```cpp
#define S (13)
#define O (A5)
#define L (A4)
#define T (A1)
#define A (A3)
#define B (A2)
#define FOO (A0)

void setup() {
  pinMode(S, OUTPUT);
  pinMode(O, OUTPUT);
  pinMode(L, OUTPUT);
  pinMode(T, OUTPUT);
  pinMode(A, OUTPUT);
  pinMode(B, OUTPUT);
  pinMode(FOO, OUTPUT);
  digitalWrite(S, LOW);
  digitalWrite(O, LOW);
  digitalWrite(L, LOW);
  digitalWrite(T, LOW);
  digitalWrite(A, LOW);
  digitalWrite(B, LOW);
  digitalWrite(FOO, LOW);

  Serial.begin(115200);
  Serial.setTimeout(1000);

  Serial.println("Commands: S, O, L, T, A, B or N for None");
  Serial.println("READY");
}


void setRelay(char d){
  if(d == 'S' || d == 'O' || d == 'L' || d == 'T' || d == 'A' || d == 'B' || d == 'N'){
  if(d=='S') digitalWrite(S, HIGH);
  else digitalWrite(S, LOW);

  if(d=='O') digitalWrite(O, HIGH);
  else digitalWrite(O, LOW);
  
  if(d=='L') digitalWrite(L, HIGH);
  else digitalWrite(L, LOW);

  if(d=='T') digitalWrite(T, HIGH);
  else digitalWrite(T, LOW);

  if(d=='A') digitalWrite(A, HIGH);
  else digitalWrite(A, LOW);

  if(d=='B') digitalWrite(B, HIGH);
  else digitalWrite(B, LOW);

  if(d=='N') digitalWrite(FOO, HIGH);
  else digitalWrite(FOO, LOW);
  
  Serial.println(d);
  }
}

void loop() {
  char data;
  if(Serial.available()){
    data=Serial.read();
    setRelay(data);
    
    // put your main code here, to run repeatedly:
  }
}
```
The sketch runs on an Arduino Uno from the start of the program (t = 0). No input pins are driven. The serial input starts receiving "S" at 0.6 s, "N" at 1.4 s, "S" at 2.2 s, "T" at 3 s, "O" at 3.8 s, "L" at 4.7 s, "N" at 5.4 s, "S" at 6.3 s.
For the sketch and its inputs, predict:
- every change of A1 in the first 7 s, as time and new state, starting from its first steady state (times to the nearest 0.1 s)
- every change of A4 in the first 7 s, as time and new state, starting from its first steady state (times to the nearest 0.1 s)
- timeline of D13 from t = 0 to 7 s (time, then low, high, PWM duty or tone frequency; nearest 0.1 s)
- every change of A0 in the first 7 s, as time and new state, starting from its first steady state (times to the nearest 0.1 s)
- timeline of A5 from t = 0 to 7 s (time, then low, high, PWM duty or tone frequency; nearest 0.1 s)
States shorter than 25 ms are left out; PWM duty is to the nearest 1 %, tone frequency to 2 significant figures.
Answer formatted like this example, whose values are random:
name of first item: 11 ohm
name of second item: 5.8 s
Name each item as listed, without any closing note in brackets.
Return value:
every change of A1 in the first 7 s, as time and new state, starting from its first steady state: 0 s low; 3 s high; 3.8 s low
every change of A4 in the first 7 s, as time and new state, starting from its first steady state: 0 s low; 4.7 s high; 5.4 s low
timeline of D13 from t = 0 to 7 s: 0 s low; 0.6 s high; 1.4 s low; 2.2 s high; 3 s low; 6.3 s high
every change of A0 in the first 7 s, as time and new state, starting from its first steady state: 0 s low; 1.4 s high; 2.2 s low; 5.4 s high; 6.3 s low
timeline of A5 from t = 0 to 7 s: 0 s low; 3.8 s high; 4.7 s low
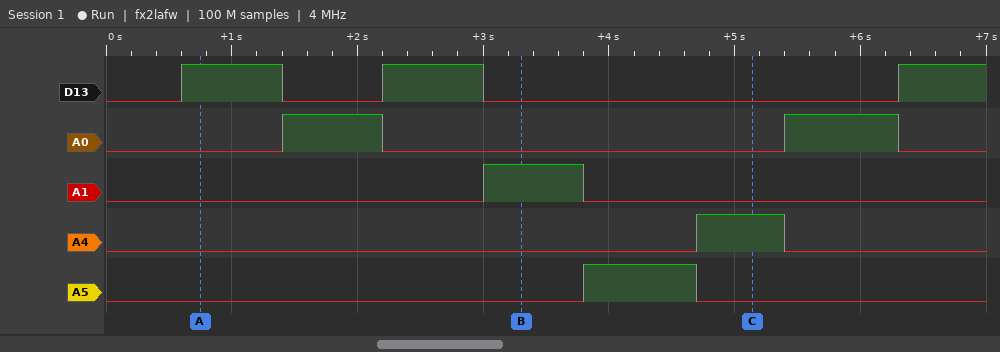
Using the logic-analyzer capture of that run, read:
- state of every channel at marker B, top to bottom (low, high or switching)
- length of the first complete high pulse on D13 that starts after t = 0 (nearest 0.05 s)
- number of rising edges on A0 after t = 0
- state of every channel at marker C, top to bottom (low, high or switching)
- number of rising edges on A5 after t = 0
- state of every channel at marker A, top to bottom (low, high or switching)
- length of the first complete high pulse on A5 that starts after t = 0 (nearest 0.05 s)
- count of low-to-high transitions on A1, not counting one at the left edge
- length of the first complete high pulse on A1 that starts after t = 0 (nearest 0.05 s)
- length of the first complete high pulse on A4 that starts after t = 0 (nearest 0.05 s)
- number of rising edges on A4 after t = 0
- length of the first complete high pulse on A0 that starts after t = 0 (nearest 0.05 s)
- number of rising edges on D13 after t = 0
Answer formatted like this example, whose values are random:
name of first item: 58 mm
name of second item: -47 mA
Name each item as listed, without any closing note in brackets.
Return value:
state of every channel at marker B, top to bottom: D13 low, A0 low, A1 high, A4 low, A5 low
length of the first complete high pulse on D13 that starts after t = 0: 0.80 s
number of rising edges on A0 after t = 0: 2
state of every channel at marker C, top to bottom: D13 low, A0 low, A1 low, A4 high, A5 low
number of rising edges on A5 after t = 0: 1
state of every channel at marker A, top to bottom: D13 high, A0 low, A1 low, A4 low, A5 low
length of the first complete high pulse on A5 that starts after t = 0: 0.90 s
count of low-to-high transitions on A1, not counting one at the left edge: 1
length of the first complete high pulse on A1 that starts after t = 0: 0.80 s
length of the first complete high pulse on A4 that starts after t = 0: 0.70 s
number of rising edges on A4 after t = 0: 1
length of the first complete high pulse on A0 that starts after t = 0: 0.80 s
number of rising edges on D13 after t = 0: 3
